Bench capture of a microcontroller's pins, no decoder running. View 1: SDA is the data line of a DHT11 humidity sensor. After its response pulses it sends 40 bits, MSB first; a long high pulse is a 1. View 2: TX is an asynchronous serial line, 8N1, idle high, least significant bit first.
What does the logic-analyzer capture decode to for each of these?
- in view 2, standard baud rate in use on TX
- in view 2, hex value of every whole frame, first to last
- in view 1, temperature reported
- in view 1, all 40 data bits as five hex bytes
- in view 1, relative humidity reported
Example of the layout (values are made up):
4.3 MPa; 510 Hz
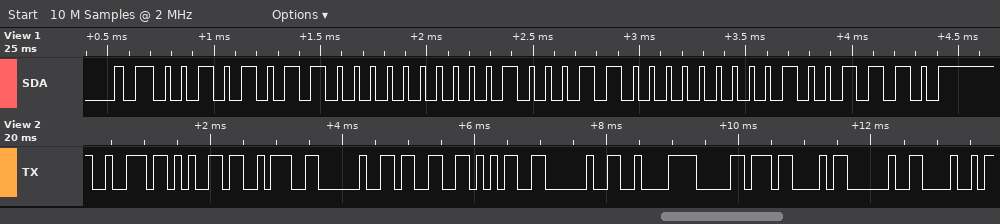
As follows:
9600 baud; 72 65 3A 20 33 35 20 C2 B0 43 20 48; 35.0 °C; 2B 00 23 00 4E; 43 %
